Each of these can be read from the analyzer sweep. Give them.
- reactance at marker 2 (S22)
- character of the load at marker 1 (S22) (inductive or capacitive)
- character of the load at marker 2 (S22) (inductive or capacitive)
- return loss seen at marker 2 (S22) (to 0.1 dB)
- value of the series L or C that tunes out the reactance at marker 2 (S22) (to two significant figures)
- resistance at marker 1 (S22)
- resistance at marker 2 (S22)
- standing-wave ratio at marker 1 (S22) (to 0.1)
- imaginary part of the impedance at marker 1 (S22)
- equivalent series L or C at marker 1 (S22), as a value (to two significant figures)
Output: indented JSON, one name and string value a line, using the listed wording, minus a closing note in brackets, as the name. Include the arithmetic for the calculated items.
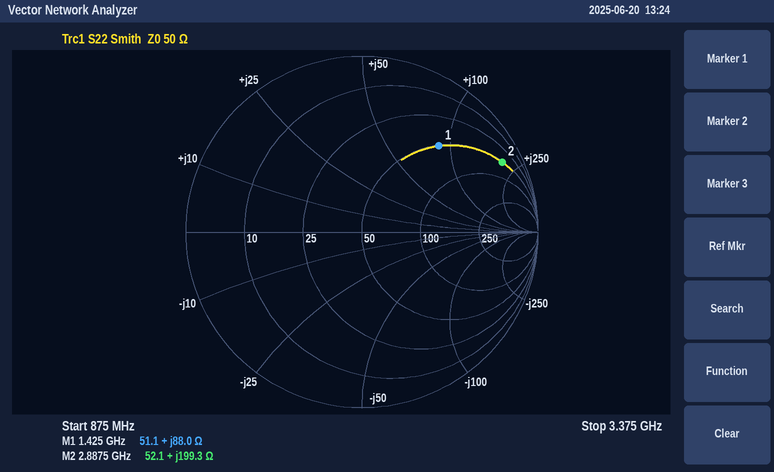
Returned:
{
  "reactance at marker 2": "+199.3 Ω",
  "character of the load at marker 1 (S22)": "inductive",
  "character of the load at marker 2 (S22)": "inductive",
  "return loss seen at marker 2 (S22)": "1.0 dB",
  "value of the series L or C that tunes out the reactance at marker 2 (S22)": "C = 1/(2π × 2.8875 GHz × 199.3 Ω) ≈ 277 fF, so 280 fF to two significant figures",
  "resistance at marker 1": "51.1 Ω",
  "resistance at marker 2": "52.1 Ω",
  "standing-wave ratio at marker 1 (S22)": "4.8",
  "imaginary part of the impedance at marker 1": "+88.0 Ω",
  "equivalent series L or C at marker 1 (S22), as a value": "L = 88 Ω/(2π × 1.425 GHz) ≈ 9.8 nH"
}
